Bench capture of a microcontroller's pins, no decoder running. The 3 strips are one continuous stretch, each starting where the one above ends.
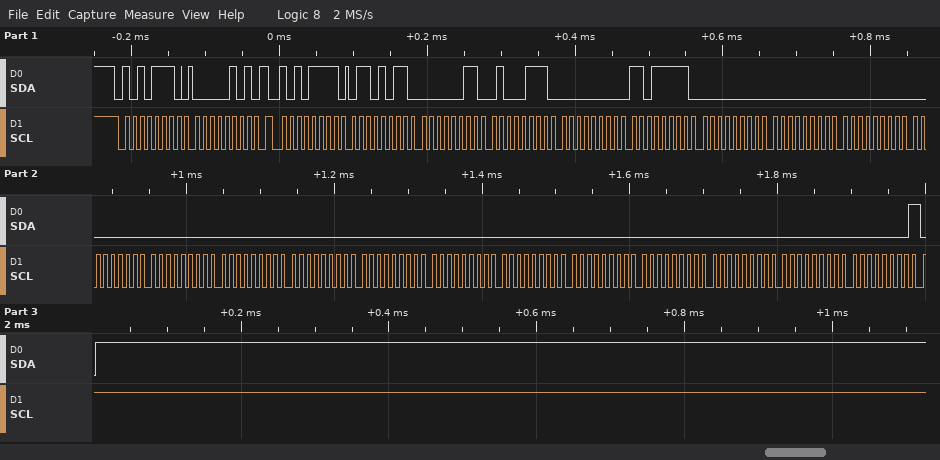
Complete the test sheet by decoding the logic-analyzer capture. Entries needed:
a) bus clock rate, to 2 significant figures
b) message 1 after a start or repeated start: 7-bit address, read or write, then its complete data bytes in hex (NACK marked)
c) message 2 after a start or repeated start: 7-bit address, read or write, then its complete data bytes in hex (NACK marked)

100 kHz
0x57 write: 05
0x57 read: 6B 03 47 00 DF 00 00 00 00 00 00 00 00 00 00 00 00 00 00 00 NACK
